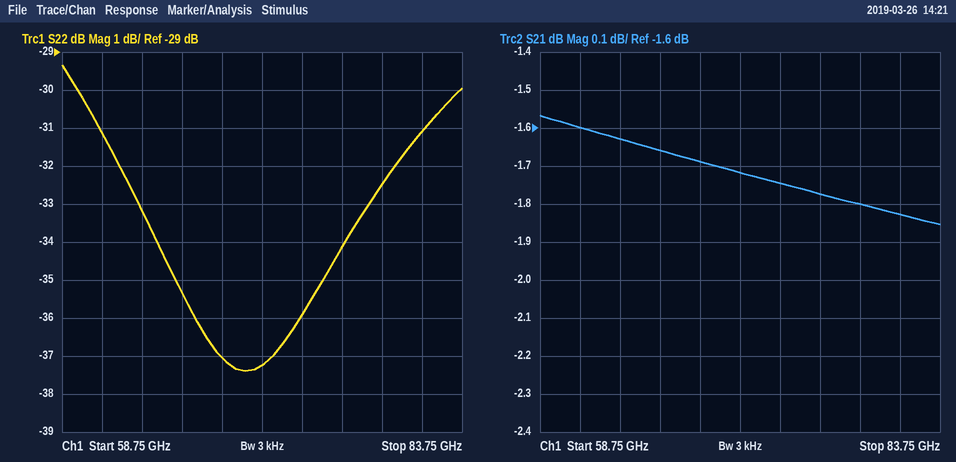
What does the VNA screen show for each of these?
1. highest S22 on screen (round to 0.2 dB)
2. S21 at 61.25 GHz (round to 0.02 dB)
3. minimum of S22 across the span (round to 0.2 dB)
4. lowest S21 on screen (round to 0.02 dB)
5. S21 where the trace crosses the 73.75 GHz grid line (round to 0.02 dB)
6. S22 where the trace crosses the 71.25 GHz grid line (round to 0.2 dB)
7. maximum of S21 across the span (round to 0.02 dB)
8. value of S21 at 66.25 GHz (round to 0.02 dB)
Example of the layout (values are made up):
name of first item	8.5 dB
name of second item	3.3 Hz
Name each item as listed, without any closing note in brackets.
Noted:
highest S22 on screen	-29.4 dB
S21 at 61.25 GHz	-1.60 dB
minimum of S22 across the span	-37.4 dB
lowest S21 on screen	-1.86 dB
S21 where the trace crosses the 73.75 GHz grid line	-1.74 dB
S22 where the trace crosses the 71.25 GHz grid line	-37.2 dB
maximum of S21 across the span	-1.56 dB
value of S21 at 66.25 GHz	-1.66 dB
